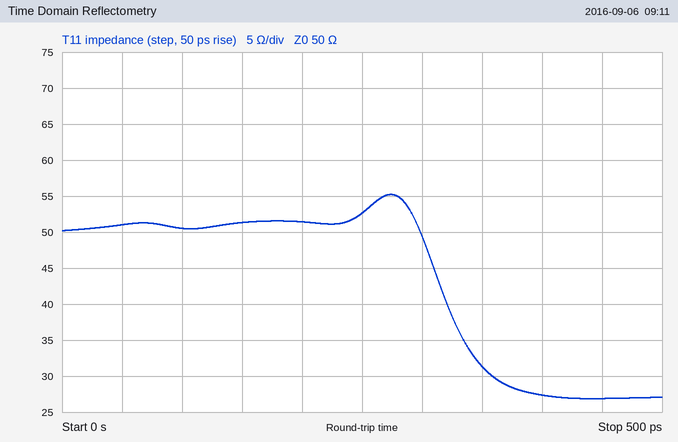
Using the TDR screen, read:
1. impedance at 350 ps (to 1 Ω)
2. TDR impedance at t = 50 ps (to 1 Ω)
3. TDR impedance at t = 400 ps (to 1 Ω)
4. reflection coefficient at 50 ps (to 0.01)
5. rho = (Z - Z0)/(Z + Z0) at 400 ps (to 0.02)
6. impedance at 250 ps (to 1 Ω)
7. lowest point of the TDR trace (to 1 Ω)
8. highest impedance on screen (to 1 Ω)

31 Ω
51 Ω
27 Ω
+0.01
-0.30
53 Ω
27 Ω
55 Ω
